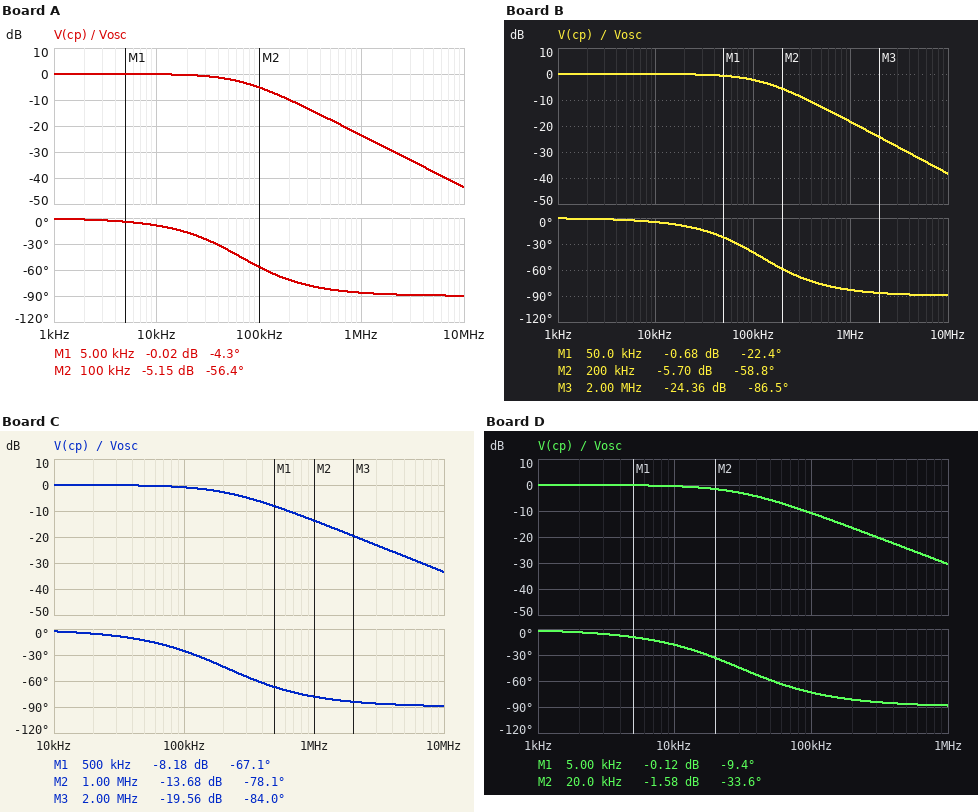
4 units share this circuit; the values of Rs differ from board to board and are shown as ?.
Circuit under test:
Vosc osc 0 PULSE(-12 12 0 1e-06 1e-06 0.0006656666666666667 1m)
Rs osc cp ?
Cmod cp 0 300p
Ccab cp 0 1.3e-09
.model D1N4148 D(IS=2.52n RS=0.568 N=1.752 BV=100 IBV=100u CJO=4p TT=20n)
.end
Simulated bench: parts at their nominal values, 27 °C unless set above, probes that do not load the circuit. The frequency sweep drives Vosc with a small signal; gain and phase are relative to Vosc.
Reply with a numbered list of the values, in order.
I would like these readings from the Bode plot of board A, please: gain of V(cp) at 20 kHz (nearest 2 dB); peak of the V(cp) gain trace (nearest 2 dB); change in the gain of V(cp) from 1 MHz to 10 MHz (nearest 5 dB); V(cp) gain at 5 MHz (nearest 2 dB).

1. 0 dB
2. 0 dB
3. -20 dB
4. -38 dB
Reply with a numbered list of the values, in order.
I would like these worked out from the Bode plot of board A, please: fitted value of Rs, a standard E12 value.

1. 1.5 kΩ
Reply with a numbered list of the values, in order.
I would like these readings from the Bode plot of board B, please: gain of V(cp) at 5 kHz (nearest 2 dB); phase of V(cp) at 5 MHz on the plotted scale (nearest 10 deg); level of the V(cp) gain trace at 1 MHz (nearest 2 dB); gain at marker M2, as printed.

1. 0 dB
2. -90 deg
3. -18 dB
4. -5.70 dB
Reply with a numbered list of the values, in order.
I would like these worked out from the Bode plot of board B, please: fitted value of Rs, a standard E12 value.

1. 820 Ω
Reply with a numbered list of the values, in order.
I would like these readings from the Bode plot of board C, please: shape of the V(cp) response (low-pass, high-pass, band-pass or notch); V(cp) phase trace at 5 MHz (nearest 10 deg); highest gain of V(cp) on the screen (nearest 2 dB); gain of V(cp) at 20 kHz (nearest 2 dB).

1. low-pass
2. -90 deg
3. 0 dB
4. 0 dB
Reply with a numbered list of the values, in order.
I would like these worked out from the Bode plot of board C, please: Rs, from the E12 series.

1. 470 Ω
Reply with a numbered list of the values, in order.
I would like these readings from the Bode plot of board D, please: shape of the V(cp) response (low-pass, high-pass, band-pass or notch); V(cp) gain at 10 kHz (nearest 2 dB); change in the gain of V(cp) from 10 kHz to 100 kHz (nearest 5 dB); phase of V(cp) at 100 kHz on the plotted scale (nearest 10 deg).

1. low-pass
2. 0 dB
3. -10 dB
4. -70 deg
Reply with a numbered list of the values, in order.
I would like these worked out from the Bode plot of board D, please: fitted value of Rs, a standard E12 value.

1. 3.3 kΩ
